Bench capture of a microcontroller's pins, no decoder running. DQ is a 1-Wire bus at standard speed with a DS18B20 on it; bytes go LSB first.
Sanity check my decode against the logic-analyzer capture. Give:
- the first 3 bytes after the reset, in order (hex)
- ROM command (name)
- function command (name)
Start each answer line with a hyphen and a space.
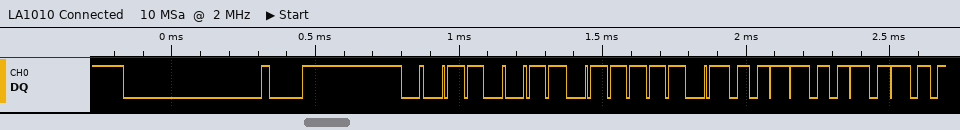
- CC BE 4C
- Skip ROM
- Read Scratchpad
